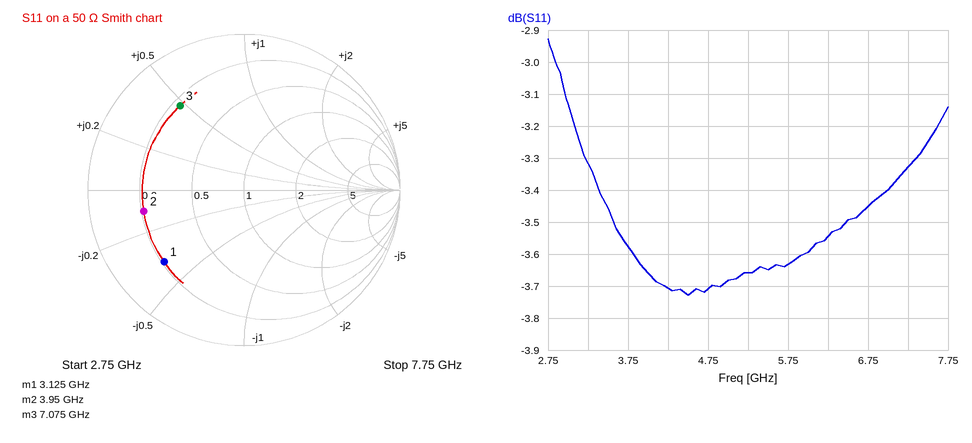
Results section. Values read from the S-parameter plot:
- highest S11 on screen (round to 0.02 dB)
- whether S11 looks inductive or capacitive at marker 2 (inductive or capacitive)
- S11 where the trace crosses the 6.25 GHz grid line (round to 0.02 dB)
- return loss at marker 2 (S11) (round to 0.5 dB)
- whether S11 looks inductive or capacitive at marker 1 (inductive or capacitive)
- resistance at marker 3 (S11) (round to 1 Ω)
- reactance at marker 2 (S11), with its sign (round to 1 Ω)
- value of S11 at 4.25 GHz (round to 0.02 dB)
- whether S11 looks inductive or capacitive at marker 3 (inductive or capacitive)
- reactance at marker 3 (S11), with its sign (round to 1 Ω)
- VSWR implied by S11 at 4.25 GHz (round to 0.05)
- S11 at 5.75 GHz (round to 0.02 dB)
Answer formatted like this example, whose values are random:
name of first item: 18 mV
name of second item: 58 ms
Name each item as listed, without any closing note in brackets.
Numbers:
highest S11 on screen: -2.92 dB
whether S11 looks inductive or capacitive at marker 2: capacitive
S11 where the trace crosses the 6.25 GHz grid line: -3.54 dB
return loss at marker 2 (S11): 3.5 dB
whether S11 looks inductive or capacitive at marker 1: capacitive
resistance at marker 3 (S11): 12 Ω
reactance at marker 2 (S11), with its sign: -5 Ω
value of S11 at 4.25 GHz: -3.70 dB
whether S11 looks inductive or capacitive at marker 3: inductive
reactance at marker 3 (S11), with its sign: +24 Ω
VSWR implied by S11 at 4.25 GHz: 4.75
S11 at 5.75 GHz: -3.64 dB
